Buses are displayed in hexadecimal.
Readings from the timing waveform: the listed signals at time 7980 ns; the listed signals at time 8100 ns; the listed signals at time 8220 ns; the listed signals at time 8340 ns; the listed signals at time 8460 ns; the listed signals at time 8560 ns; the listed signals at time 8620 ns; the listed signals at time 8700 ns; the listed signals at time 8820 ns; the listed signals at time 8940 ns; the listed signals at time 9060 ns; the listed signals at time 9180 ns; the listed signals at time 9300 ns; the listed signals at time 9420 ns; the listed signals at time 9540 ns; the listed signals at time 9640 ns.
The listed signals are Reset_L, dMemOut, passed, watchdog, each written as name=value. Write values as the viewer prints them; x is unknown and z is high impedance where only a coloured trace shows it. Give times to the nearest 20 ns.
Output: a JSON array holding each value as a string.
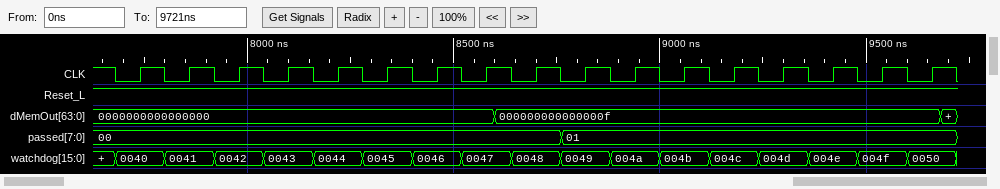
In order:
["Reset_L=1, dMemOut=0000000000000000, passed=00, watchdog=0042", "Reset_L=1, dMemOut=0000000000000000, passed=00, watchdog=0043", "Reset_L=1, dMemOut=0000000000000000, passed=00, watchdog=0044", "Reset_L=1, dMemOut=0000000000000000, passed=00, watchdog=0045", "Reset_L=1, dMemOut=0000000000000000, passed=00, watchdog=0046", "Reset_L=1, dMemOut=0000000000000000, passed=00, watchdog=0047", "Reset_L=1, dMemOut=000000000000000f, passed=00, watchdog=0047", "Reset_L=1, dMemOut=000000000000000f, passed=00, watchdog=0048", "Reset_L=1, dMemOut=000000000000000f, passed=01, watchdog=0049", "Reset_L=1, dMemOut=000000000000000f, passed=01, watchdog=004a", "Reset_L=1, dMemOut=000000000000000f, passed=01, watchdog=004b", "Reset_L=1, dMemOut=000000000000000f, passed=01, watchdog=004c", "Reset_L=1, dMemOut=000000000000000f, passed=01, watchdog=004d", "Reset_L=1, dMemOut=000000000000000f, passed=01, watchdog=004e", "Reset_L=1, dMemOut=000000000000000f, passed=01, watchdog=004f", "Reset_L=1, dMemOut=000000000000000f, passed=01, watchdog=0050"]
